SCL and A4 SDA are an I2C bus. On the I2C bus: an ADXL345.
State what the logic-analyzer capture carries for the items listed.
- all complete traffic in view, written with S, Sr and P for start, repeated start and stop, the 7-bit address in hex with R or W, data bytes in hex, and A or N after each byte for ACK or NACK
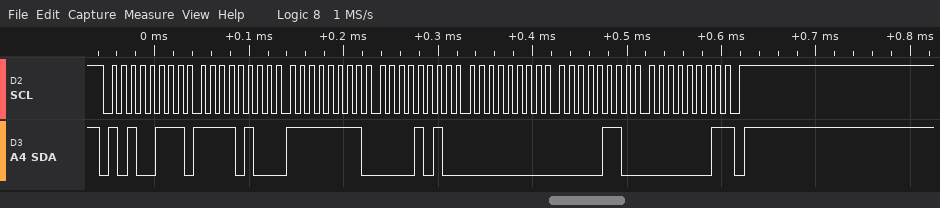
S 53R A F4 A FF A 0A A 00 A 06 A 01 N P
